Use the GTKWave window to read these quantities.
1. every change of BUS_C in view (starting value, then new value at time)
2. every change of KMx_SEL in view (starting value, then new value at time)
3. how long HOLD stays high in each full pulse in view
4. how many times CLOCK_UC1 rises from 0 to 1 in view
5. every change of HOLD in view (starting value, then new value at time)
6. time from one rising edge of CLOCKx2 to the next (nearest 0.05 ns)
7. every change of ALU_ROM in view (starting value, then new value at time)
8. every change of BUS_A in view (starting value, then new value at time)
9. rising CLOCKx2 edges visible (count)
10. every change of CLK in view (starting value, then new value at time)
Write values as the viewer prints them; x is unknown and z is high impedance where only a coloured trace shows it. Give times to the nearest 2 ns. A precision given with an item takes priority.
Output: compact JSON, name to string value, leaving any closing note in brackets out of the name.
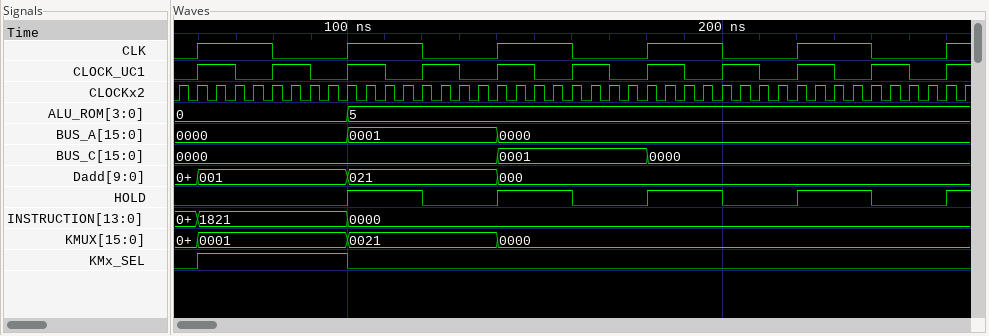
{"every change of BUS_C in view": "0000, 0001 at 140 ns, 0000 at 180 ns", "every change of KMx_SEL in view": "0, 1 at 60 ns, 0 at 100 ns", "how long HOLD stays high in each full pulse in view": "20 ns, 20 ns, 20 ns, 20 ns", "how many times CLOCK_UC1 rises from 0 to 1 in view": "11", "every change of HOLD in view": "0, 1 at 100 ns, 0 at 120 ns, 1 at 140 ns, 0 at 160 ns, 1 at 180 ns, 0 at 200 ns, 1 at 220 ns, 0 at 240 ns, 1 at 260 ns", "time from one rising edge of CLOCKx2 to the next": "5 ns", "every change of ALU_ROM in view": "0, 5 at 100 ns", "every change of BUS_A in view": "0000, 0001 at 100 ns, 0000 at 140 ns", "rising CLOCKx2 edges visible": "43", "every change of CLK in view": "0, 1 at 60 ns, 0 at 80 ns, 1 at 100 ns, 0 at 120 ns, 1 at 140 ns, 0 at 160 ns, 1 at 180 ns, 0 at 200 ns, 1 at 220 ns, 0 at 240 ns, 1 at 260 ns"}
